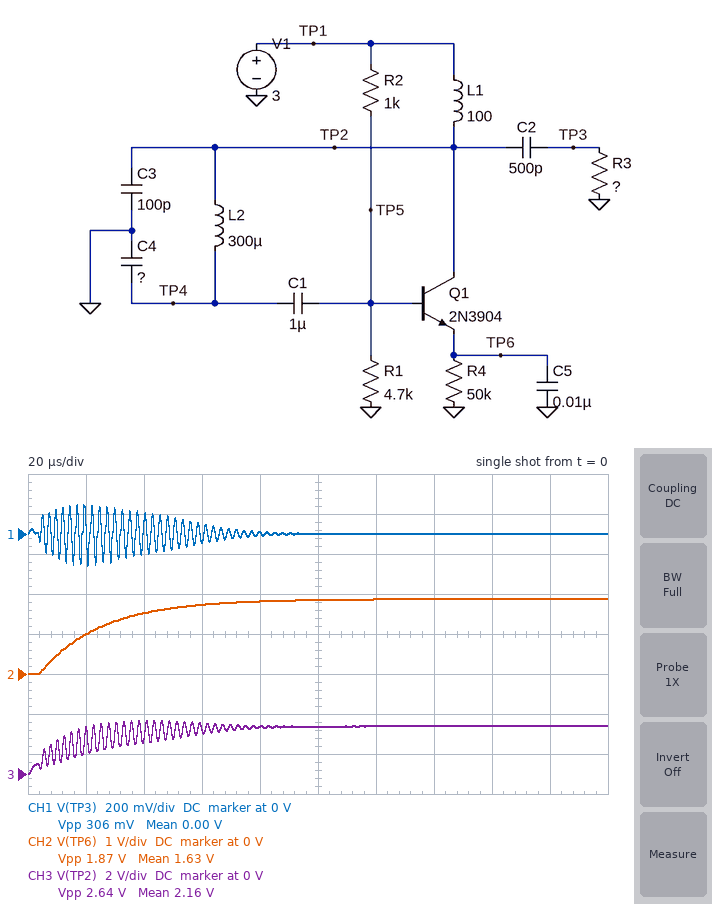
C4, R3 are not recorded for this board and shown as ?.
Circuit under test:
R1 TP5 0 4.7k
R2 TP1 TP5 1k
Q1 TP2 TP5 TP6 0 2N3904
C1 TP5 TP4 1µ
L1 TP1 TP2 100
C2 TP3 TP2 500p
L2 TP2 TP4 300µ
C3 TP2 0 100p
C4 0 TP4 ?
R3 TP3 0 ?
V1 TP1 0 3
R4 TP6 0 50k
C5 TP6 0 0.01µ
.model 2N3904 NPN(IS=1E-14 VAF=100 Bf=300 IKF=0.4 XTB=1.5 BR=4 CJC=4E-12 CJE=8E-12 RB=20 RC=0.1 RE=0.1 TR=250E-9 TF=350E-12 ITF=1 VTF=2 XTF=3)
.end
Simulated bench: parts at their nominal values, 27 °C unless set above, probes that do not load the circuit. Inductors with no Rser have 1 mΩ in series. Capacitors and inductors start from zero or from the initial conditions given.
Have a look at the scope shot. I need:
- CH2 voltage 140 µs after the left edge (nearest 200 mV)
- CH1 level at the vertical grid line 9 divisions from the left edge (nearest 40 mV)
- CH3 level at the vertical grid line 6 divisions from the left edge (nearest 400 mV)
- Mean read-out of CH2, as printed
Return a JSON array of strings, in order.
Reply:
["1.8 V", "0 V", "2.4 V", "1.63 V"]
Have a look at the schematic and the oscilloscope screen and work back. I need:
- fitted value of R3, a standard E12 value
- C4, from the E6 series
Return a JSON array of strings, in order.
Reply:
["150 Ω", "15 nF"]
